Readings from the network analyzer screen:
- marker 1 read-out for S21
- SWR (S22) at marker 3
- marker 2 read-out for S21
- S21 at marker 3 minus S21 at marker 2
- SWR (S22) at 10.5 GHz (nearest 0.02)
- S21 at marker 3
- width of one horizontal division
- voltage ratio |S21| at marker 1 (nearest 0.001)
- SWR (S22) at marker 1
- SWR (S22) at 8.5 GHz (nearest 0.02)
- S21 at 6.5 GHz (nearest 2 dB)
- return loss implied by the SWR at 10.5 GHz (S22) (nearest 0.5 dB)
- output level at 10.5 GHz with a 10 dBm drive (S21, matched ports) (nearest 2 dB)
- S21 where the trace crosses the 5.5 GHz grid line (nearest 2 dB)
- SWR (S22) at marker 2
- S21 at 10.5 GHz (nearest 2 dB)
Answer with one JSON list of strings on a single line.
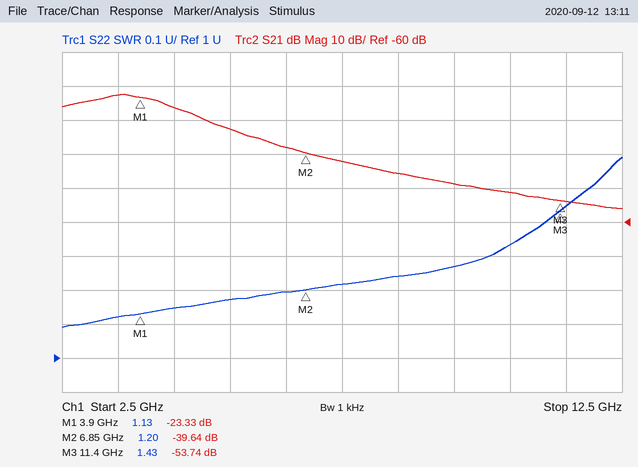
["-23.33 dB", "1.43", "-39.64 dB", "-14.10 dB", "1.34", "-53.74 dB", "1 GHz", "0.068", "1.13", "1.24", "-38 dB", "17.0 dB", "-42 dBm", "-32 dB", "1.20", "-52 dB"]
